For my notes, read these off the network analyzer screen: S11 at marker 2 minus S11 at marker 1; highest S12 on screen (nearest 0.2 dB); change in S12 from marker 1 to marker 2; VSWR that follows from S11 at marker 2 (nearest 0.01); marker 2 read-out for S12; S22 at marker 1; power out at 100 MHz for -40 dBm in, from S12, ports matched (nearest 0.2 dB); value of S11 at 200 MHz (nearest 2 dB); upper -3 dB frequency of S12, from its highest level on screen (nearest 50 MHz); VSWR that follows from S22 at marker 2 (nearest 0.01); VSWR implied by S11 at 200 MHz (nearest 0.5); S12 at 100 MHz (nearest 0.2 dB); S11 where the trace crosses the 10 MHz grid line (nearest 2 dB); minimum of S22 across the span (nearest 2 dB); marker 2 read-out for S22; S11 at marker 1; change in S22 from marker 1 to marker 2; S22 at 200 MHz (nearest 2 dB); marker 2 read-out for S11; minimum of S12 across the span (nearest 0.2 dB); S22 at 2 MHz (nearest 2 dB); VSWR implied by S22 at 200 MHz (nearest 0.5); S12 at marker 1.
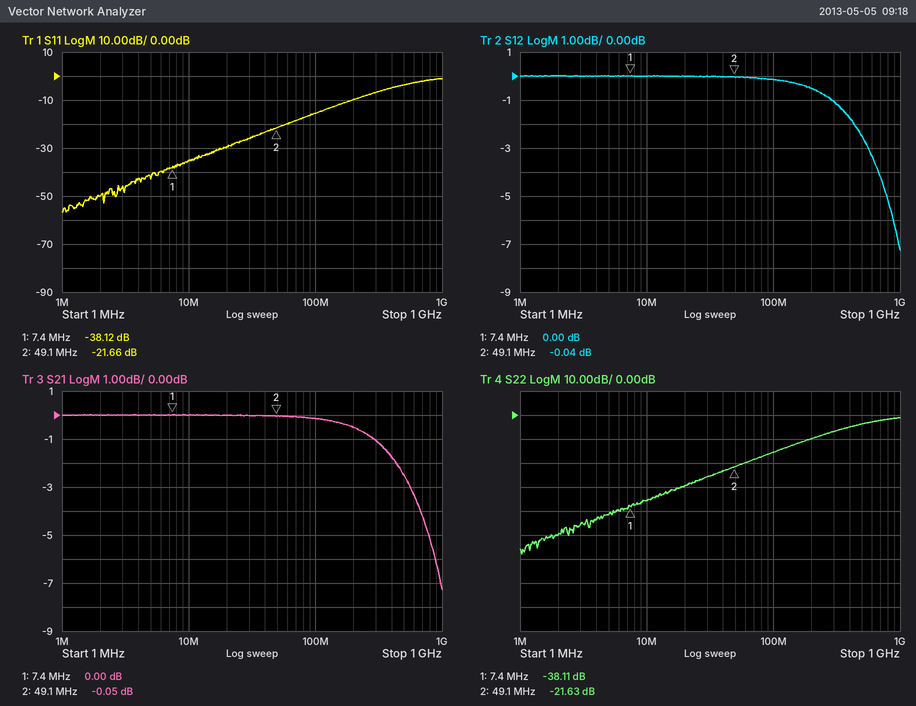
16.46 dB
0.0 dB
-0.04 dB
1.18
-0.04 dB
-38.11 dB
-40.2 dBm
-10 dB
550 MHz
1.18
2.0
-0.2 dB
-36 dB
-58 dB
-21.63 dB
-38.12 dB
16.48 dB
-10 dB
-21.66 dB
-7.2 dB
-50 dB
2.0
0.00 dB
